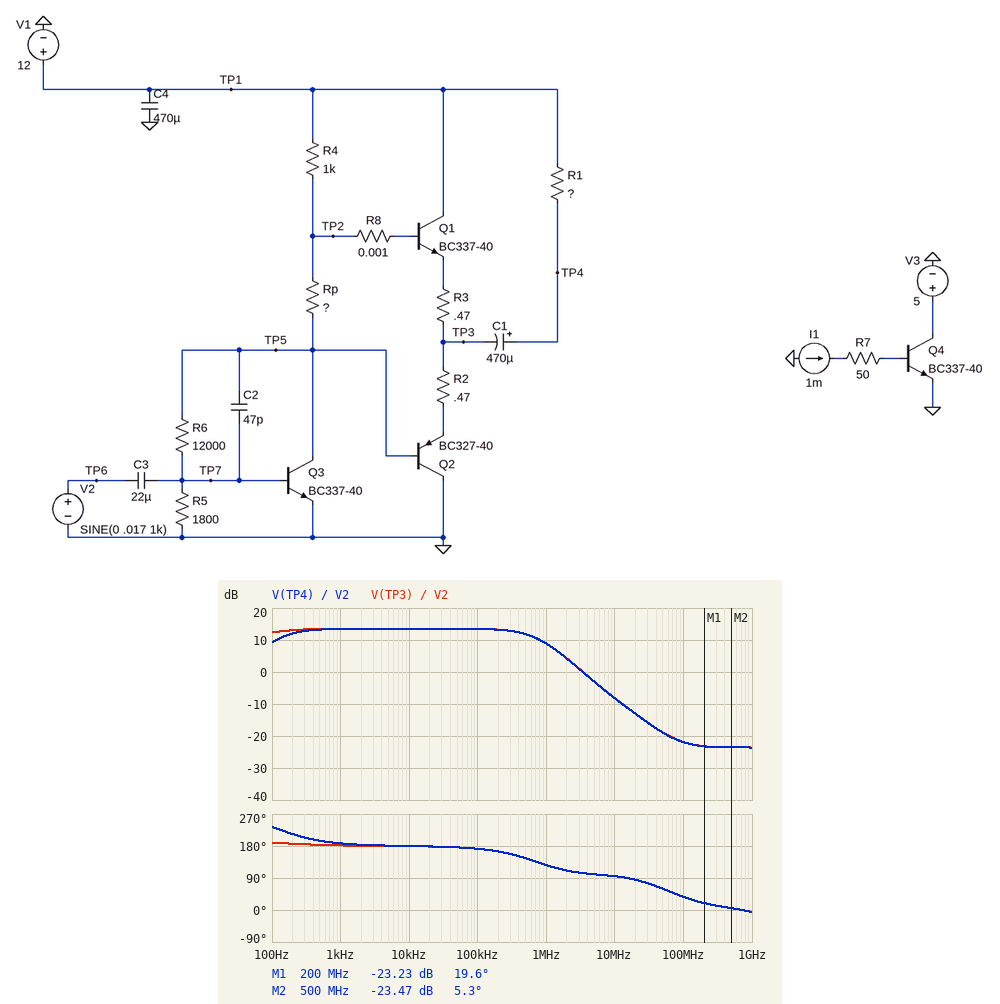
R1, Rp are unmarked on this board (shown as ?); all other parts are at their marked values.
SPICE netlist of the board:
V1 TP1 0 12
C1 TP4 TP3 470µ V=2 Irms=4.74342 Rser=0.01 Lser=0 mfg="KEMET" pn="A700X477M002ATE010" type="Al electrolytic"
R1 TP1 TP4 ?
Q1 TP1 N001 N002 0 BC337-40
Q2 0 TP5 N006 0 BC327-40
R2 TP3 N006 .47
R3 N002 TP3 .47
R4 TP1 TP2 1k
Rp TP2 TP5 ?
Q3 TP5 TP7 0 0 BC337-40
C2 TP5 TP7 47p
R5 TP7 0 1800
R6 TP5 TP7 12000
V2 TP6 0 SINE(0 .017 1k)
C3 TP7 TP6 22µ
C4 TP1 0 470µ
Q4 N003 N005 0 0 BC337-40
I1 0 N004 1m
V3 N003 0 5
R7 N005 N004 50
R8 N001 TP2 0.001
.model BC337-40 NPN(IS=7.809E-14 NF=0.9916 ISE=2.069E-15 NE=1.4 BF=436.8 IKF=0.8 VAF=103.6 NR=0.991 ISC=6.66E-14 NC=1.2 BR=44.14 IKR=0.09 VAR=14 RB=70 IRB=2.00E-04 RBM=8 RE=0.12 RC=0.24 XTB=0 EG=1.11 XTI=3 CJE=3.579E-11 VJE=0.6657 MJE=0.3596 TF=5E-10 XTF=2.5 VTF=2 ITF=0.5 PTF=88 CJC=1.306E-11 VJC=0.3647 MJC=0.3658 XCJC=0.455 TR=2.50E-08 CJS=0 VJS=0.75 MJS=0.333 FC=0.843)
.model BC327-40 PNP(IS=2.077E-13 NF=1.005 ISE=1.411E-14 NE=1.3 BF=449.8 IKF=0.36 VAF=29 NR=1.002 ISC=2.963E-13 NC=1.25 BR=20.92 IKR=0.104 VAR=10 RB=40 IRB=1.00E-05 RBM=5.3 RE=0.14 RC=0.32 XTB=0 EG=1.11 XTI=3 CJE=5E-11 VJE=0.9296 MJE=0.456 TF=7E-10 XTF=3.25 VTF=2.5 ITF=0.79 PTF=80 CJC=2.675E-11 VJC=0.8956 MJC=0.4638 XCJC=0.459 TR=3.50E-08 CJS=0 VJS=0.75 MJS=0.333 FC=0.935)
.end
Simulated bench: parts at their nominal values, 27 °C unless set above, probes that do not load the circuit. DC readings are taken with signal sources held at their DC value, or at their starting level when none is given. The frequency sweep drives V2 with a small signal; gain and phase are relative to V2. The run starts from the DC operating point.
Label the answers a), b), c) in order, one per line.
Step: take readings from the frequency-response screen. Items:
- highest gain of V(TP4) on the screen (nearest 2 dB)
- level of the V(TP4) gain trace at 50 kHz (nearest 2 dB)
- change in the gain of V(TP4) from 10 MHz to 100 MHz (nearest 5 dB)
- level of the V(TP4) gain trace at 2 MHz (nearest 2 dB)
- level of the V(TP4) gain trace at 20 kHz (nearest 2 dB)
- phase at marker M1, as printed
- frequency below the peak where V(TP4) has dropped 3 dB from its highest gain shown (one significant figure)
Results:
a) 14 dB
b) 14 dB
c) -15 dB
d) 4 dB
e) 14 dB
f) 19.6 deg
g) 100 Hz
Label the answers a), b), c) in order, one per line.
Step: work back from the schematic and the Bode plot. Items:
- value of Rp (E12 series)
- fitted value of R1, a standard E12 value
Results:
a) 180 Ω
b) 3.3 Ω
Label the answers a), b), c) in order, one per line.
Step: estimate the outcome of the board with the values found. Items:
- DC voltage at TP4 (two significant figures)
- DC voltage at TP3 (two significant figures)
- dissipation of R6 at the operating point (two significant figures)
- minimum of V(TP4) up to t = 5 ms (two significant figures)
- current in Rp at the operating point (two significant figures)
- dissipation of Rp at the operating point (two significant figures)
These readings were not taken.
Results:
a) 12 V
b) 5.6 V
c) 1.6 mW
d) 11 V
e) 5.9 mA
f) 6.2 mW
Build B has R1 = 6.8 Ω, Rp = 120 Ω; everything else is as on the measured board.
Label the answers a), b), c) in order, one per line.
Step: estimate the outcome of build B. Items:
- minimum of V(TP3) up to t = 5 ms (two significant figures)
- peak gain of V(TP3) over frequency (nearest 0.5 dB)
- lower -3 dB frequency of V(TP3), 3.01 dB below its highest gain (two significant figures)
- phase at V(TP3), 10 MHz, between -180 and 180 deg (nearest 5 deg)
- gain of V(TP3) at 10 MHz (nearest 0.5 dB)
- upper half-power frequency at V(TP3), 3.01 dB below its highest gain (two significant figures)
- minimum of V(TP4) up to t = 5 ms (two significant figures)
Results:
a) 3.3 V
b) -3.0 dB
c) 730 kHz
d) 140 deg
e) -4.5 dB
f) 16 MHz
g) 9.9 V
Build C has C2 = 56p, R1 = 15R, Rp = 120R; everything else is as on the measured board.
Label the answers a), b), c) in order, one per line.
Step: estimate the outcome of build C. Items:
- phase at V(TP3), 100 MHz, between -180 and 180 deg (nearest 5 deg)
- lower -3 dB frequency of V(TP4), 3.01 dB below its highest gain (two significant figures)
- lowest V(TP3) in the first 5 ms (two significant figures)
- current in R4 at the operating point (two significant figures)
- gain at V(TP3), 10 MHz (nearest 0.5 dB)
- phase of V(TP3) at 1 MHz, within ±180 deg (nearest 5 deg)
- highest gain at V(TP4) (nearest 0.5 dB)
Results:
a) 30 deg
b) 700 kHz
c) 2.7 V
d) 6.2 mA
e) 2.0 dB
f) -150 deg
g) 3.5 dB
